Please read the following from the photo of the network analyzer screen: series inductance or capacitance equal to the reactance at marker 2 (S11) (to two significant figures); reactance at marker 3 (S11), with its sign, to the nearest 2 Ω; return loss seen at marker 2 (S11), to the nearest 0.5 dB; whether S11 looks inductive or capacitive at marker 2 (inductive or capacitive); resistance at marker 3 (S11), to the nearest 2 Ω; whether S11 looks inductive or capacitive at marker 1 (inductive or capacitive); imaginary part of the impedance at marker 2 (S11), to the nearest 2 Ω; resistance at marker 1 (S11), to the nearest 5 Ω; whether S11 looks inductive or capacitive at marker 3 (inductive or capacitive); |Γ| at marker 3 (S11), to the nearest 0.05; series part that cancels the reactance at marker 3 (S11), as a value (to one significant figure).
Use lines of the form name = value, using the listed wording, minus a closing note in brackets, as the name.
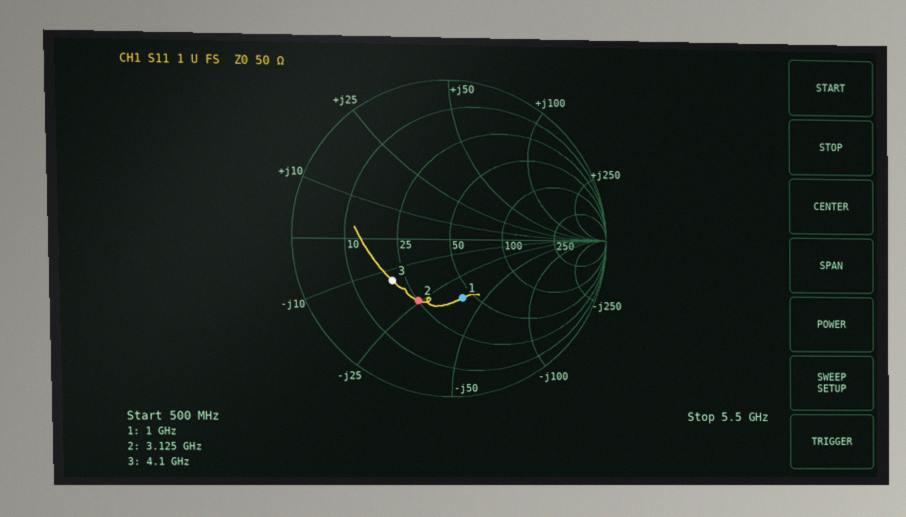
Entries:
series inductance or capacitance equal to the reactance at marker 2 (S11) = 2.1 pF
reactance at marker 3 (S11), with its sign, to the nearest 2 Ω = -14 Ω
return loss seen at marker 2 (S11), to the nearest 0.5 dB = 7.0 dB
whether S11 looks inductive or capacitive at marker 2 = capacitive
resistance at marker 3 (S11), to the nearest 2 Ω = 20 Ω
whether S11 looks inductive or capacitive at marker 1 = capacitive
imaginary part of the impedance at marker 2 (S11), to the nearest 2 Ω = -24 Ω
resistance at marker 1 (S11), to the nearest 5 Ω = 45 Ω
whether S11 looks inductive or capacitive at marker 3 = capacitive
|Γ| at marker 3 (S11), to the nearest 0.05 = 0.45
series part that cancels the reactance at marker 3 (S11), as a value = 500 pH
